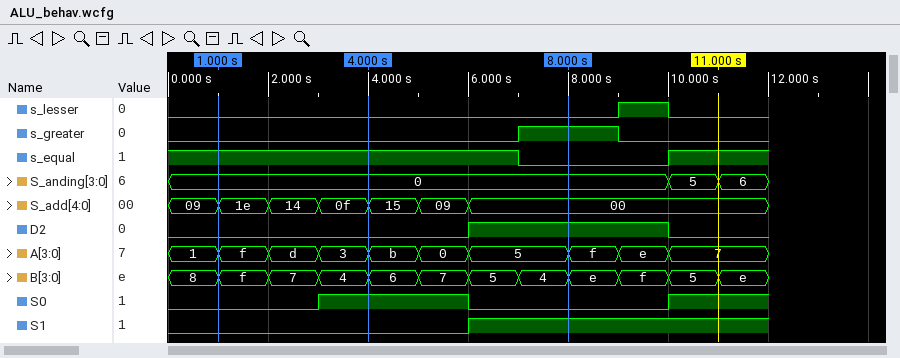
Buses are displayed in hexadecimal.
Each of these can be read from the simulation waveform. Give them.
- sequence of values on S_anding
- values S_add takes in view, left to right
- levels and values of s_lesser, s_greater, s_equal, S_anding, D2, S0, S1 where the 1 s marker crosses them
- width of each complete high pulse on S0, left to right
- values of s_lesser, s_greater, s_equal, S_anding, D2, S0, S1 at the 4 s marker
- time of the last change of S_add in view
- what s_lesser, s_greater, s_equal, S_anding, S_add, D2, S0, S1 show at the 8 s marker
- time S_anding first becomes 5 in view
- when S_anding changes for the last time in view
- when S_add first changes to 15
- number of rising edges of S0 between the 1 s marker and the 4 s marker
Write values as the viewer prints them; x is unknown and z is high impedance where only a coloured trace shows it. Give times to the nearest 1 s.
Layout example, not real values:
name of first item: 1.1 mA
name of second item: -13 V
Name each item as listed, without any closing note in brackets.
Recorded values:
sequence of values on S_anding: 0, 5, 6
values S_add takes in view, left to right: 09, 1e, 14, 0f, 15, 09, 00
levels and values of s_lesser, s_greater, s_equal, S_anding, D2, S0, S1 where the 1 s marker crosses them: s_lesser=0, s_greater=0, s_equal=1, S_anding=0, D2=0, S0=0, S1=0
width of each complete high pulse on S0, left to right: 3 s
values of s_lesser, s_greater, s_equal, S_anding, D2, S0, S1 at the 4 s marker: s_lesser=0, s_greater=0, s_equal=1, S_anding=0, D2=0, S0=1, S1=0
time of the last change of S_add in view: 6 s
what s_lesser, s_greater, s_equal, S_anding, S_add, D2, S0, S1 show at the 8 s marker: s_lesser=0, s_greater=1, s_equal=0, S_anding=0, S_add=00, D2=1, S0=0, S1=1
time S_anding first becomes 5 in view: 10 s
when S_anding changes for the last time in view: 11 s
when S_add first changes to 15: 4 s
number of rising edges of S0 between the 1 s marker and the 4 s marker: 1
